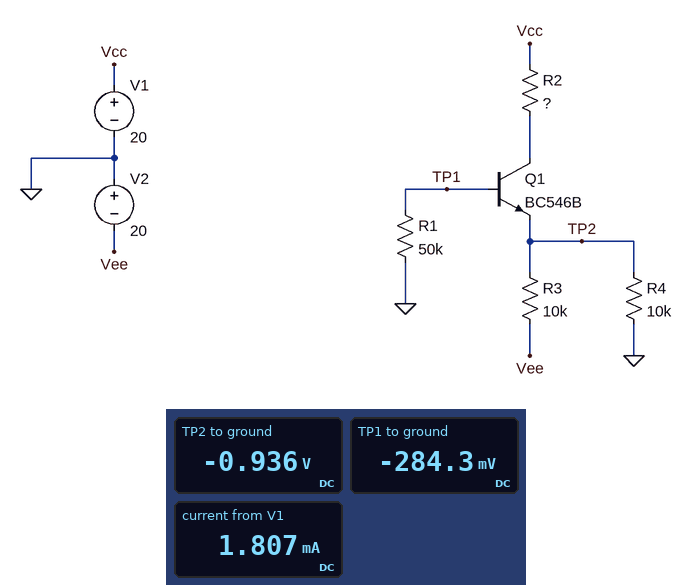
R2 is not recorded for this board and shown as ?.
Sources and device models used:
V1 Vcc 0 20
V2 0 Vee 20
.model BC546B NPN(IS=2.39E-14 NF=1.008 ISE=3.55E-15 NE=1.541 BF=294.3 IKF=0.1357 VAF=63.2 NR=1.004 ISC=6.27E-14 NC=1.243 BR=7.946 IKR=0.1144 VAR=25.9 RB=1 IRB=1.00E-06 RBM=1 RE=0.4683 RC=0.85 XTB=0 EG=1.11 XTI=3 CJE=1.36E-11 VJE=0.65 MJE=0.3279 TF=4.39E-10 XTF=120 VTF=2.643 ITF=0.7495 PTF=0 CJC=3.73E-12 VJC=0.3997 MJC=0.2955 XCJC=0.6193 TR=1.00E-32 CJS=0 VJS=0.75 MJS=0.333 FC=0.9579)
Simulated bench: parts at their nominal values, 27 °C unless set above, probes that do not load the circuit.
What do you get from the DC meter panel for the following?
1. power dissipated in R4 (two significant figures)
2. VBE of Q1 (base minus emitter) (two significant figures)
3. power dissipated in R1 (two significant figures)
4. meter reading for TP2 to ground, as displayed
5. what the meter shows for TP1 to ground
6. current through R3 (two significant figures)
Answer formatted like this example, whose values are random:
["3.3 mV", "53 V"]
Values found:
["88 µW", "650 mV", "1.6 µW", "-0.936 V", "-284.3 mV", "1.9 mA"]
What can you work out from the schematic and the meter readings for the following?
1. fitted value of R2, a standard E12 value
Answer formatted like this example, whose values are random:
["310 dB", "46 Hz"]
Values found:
["6.8 kΩ"]
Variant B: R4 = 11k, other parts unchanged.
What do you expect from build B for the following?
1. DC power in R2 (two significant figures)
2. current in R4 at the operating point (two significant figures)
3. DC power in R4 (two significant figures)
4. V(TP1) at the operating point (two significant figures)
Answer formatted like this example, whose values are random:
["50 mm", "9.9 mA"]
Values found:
["22 mW", "85 µA", "80 µW", "-290 mV"]
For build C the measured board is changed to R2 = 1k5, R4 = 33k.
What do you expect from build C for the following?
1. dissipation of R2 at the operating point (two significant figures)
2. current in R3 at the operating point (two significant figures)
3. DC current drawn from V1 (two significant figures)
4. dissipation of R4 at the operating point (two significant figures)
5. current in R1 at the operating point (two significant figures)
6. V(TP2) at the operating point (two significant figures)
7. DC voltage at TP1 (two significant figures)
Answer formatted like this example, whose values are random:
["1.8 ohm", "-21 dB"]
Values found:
["5.3 mW", "1.9 mA", "1.9 mA", "25 µW", "5.2 µA", "-910 mV", "-260 mV"]
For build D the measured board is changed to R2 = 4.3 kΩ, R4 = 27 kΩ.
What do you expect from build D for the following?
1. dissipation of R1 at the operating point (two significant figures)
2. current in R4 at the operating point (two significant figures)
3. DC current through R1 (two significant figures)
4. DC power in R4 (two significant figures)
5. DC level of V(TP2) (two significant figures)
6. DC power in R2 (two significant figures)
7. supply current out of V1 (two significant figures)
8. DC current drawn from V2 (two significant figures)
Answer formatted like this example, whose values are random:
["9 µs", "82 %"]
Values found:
["1.5 µW", "34 µA", "5.5 µA", "32 µW", "-930 mV", "15 mW", "1.9 mA", "1.9 mA"]
